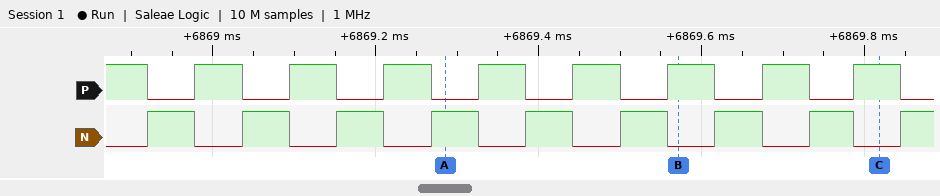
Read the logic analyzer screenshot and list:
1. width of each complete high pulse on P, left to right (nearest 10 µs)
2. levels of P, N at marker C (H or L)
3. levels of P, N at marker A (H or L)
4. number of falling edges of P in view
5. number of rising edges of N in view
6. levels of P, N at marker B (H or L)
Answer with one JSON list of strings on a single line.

["60 µs, 60 µs, 60 µs, 60 µs, 60 µs, 60 µs, 60 µs, 60 µs", "P=H, N=L", "P=L, N=H", "9", "9", "P=H, N=L"]
